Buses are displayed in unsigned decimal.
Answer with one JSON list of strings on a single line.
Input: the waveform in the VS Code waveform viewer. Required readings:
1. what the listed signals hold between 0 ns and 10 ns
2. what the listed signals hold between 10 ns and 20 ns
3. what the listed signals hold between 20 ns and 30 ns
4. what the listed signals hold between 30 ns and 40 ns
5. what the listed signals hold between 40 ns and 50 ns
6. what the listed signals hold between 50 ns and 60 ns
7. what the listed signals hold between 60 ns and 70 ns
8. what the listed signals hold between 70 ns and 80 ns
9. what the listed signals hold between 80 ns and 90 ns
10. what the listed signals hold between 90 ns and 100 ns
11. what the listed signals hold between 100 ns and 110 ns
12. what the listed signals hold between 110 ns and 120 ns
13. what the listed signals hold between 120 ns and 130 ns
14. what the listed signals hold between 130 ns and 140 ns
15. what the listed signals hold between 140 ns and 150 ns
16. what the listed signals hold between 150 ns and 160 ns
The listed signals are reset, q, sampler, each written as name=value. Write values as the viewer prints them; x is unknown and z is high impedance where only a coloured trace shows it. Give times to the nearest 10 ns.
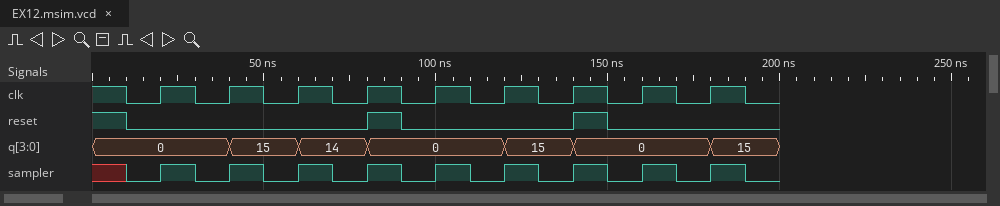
["reset=1, q=0, sampler=x", "reset=0, q=0, sampler=0", "reset=0, q=0, sampler=1", "reset=0, q=0, sampler=0", "reset=0, q=15, sampler=1", "reset=0, q=15, sampler=0", "reset=0, q=14, sampler=1", "reset=0, q=14, sampler=0", "reset=1, q=0, sampler=1", "reset=0, q=0, sampler=0", "reset=0, q=0, sampler=1", "reset=0, q=0, sampler=0", "reset=0, q=15, sampler=1", "reset=0, q=15, sampler=0", "reset=1, q=0, sampler=1", "reset=0, q=0, sampler=0"]
